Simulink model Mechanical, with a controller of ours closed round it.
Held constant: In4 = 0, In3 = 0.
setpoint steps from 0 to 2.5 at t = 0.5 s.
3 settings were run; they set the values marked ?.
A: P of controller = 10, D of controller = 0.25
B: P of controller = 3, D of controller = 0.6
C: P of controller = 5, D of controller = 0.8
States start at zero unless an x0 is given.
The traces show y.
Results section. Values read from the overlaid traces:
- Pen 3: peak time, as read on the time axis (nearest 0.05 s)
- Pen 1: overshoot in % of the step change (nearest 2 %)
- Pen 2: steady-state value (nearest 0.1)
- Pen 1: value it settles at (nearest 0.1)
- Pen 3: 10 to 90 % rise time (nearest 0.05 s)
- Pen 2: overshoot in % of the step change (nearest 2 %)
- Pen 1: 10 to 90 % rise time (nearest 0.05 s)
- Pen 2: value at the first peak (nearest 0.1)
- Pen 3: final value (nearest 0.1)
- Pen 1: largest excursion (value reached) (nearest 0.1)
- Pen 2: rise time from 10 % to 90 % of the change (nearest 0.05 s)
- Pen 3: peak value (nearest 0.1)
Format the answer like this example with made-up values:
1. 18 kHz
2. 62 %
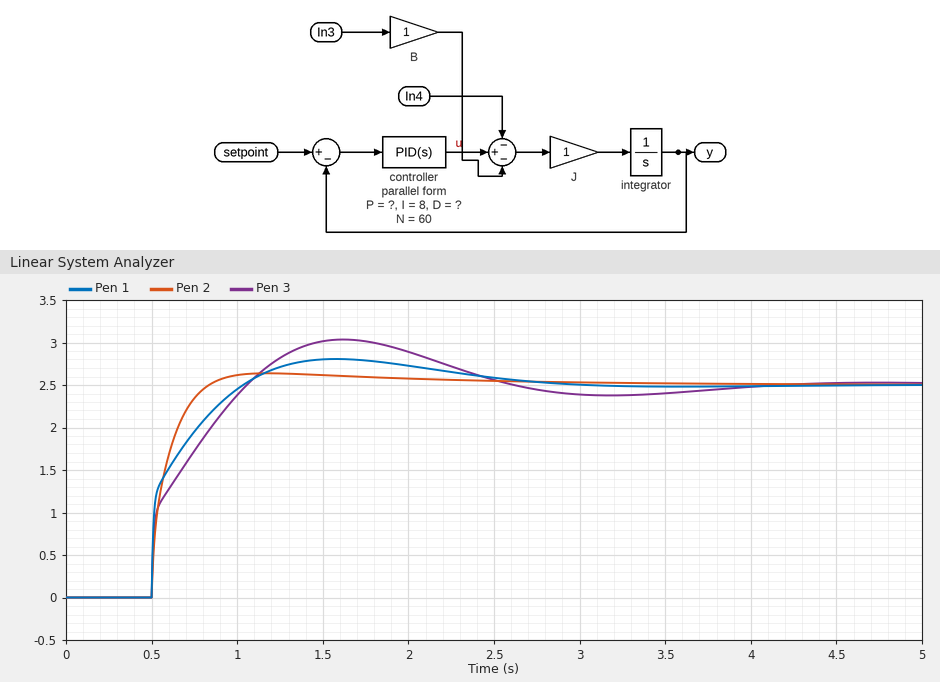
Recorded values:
1. 1.60 s
2. 12 %
3. 2.5
4. 2.5
5. 0.45 s
6. 6 %
7. 0.40 s
8. 2.6
9. 2.5
10. 2.8
11. 0.20 s
12. 3.0
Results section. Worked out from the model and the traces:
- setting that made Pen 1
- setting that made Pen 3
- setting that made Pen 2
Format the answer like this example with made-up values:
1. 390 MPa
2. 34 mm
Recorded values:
1. C
2. B
3. A
